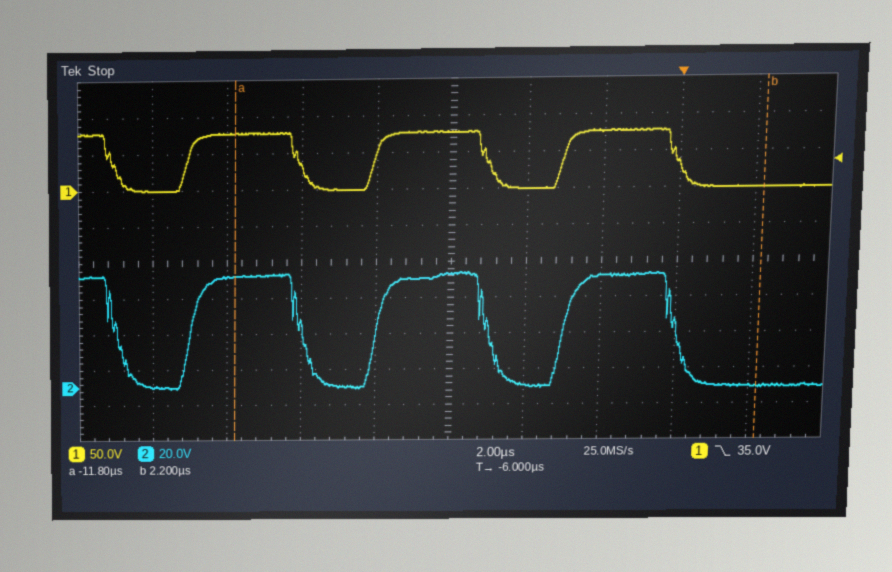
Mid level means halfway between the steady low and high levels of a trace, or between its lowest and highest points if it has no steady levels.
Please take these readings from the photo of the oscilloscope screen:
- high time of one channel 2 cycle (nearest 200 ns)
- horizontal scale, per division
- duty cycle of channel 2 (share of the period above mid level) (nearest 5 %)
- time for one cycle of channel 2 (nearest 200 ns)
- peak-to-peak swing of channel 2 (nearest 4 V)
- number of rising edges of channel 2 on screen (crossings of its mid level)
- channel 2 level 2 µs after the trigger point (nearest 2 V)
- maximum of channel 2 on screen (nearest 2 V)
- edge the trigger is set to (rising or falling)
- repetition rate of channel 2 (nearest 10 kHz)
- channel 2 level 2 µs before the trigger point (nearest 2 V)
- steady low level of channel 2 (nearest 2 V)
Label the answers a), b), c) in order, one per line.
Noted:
a) 3.0 µs
b) 2 µs
c) 60 %
d) 5.0 µs
e) 64 V
f) 3
g) 0 V
h) 64 V
i) falling
j) 200 kHz
k) 62 V
l) 0 V
